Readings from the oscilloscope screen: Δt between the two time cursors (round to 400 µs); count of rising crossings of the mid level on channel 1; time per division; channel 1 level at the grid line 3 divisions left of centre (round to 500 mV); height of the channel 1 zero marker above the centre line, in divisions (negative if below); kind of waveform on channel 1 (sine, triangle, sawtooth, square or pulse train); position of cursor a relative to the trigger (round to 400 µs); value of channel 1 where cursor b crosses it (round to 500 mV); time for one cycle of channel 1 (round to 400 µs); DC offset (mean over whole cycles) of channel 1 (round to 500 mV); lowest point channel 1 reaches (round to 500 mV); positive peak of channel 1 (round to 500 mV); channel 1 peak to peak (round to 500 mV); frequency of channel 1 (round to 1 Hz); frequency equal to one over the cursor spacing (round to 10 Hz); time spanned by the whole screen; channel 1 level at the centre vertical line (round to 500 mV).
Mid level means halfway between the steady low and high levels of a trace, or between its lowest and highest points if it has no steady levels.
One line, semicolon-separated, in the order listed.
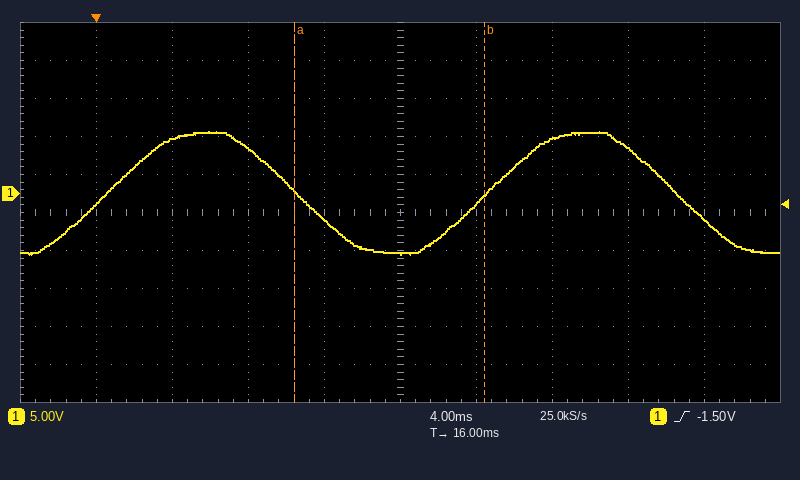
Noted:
10.0 ms; 2; 4 ms; 7.0 V; +0.5 div; sine; +10.4 ms; 0.0 V; 20.0 ms; 0.0 V; -8.0 V; 8.0 V; 16.0 V; 50 Hz; 100 Hz; 40 ms; -8.0 V
